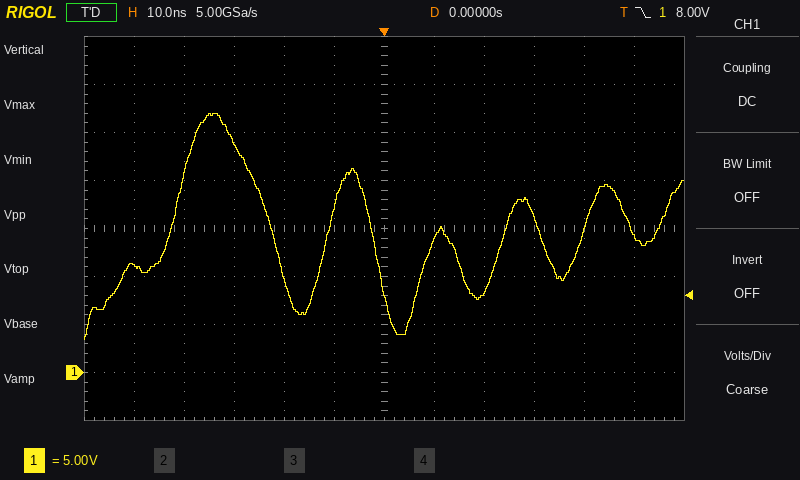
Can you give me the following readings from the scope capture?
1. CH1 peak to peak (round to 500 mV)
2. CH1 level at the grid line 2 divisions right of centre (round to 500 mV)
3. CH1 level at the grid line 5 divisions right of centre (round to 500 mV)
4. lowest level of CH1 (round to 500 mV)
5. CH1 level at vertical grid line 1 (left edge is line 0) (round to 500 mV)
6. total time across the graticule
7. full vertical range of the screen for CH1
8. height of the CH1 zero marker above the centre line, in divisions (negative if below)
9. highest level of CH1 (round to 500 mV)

23.5 V
8.5 V
14.5 V
3.5 V
11.0 V
120 ns
40 V
-3.0 div
27.0 V
